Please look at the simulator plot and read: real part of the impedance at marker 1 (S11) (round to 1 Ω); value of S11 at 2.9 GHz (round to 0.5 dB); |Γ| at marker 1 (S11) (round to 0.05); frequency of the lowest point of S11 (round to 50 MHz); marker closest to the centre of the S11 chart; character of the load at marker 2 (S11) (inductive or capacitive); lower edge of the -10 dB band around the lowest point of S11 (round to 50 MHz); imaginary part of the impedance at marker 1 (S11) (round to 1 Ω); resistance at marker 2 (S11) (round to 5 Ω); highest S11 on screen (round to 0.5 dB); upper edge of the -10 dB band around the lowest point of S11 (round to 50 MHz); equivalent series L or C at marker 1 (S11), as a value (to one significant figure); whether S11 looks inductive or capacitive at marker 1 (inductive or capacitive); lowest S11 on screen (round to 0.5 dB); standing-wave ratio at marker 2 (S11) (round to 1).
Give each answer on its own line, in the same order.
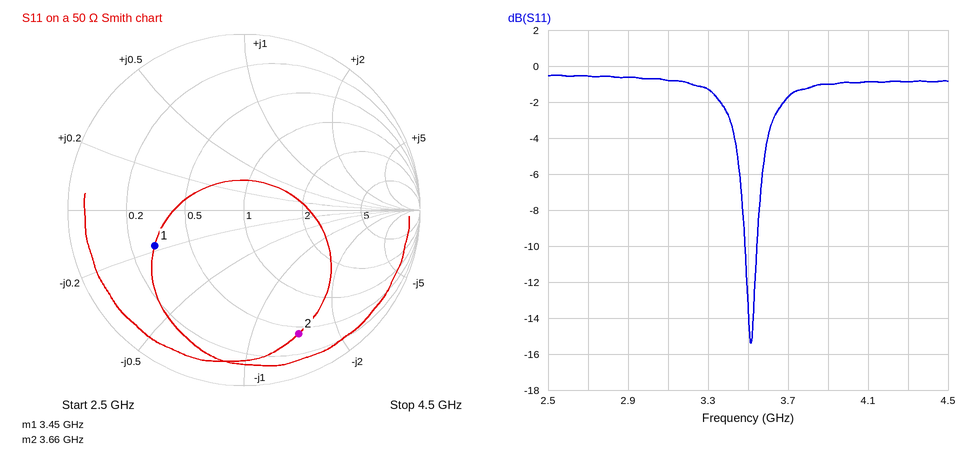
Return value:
15 Ω
-0.5 dB
0.55
3.50 GHz
marker 1
capacitive
3.50 GHz
-9 Ω
20 Ω
-0.5 dB
3.55 GHz
5 pF
capacitive
-15.5 dB
8
